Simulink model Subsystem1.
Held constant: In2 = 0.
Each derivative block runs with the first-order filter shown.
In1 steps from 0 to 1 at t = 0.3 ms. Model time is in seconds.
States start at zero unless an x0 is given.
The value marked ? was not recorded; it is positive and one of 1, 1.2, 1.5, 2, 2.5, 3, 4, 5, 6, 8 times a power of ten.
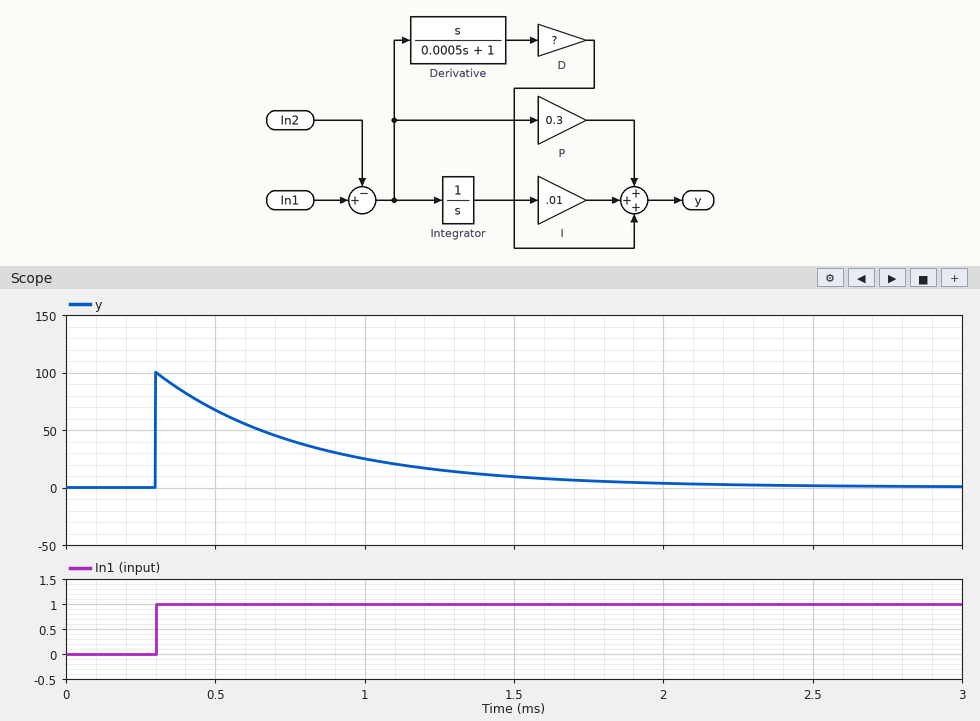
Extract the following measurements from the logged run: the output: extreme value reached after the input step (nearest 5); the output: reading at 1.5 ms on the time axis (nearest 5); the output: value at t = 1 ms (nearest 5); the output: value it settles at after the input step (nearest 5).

100
10
25
0
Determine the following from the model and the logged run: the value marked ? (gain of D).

0.05
